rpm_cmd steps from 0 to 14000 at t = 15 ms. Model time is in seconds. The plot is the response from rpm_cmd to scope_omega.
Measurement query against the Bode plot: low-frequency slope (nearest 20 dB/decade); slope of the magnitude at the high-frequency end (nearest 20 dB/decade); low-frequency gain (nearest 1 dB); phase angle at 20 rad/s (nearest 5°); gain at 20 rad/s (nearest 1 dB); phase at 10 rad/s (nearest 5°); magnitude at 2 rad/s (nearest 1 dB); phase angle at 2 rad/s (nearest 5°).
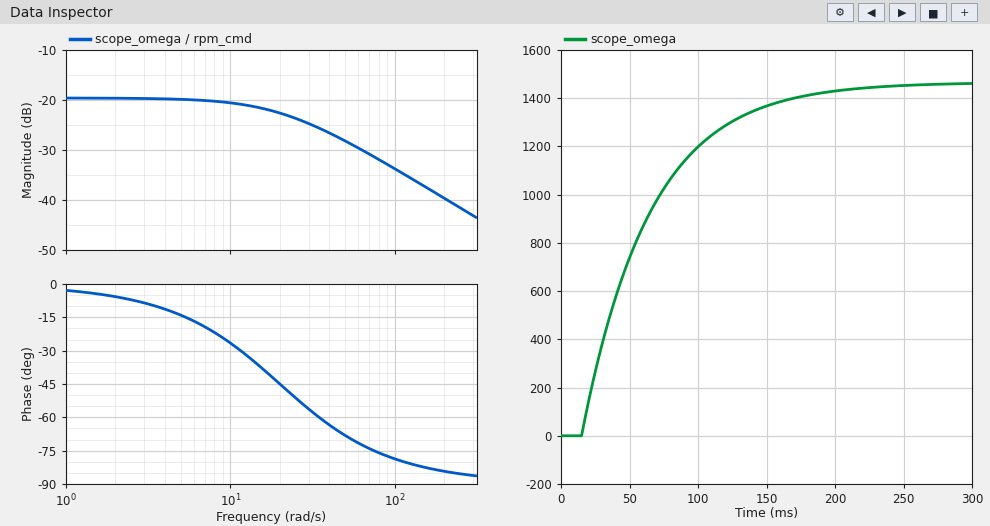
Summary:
0 dB/decade
-20 dB/decade
-20 dB
-45°
-23 dB
-25°
-20 dB
-5°
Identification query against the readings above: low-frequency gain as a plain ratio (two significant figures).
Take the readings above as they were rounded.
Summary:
0.10
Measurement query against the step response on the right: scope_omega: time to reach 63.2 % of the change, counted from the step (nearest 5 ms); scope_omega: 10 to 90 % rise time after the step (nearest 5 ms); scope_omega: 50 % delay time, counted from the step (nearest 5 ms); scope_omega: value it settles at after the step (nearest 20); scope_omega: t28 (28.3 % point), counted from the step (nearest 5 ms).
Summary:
50 ms
110 ms
35 ms
1460
15 ms
